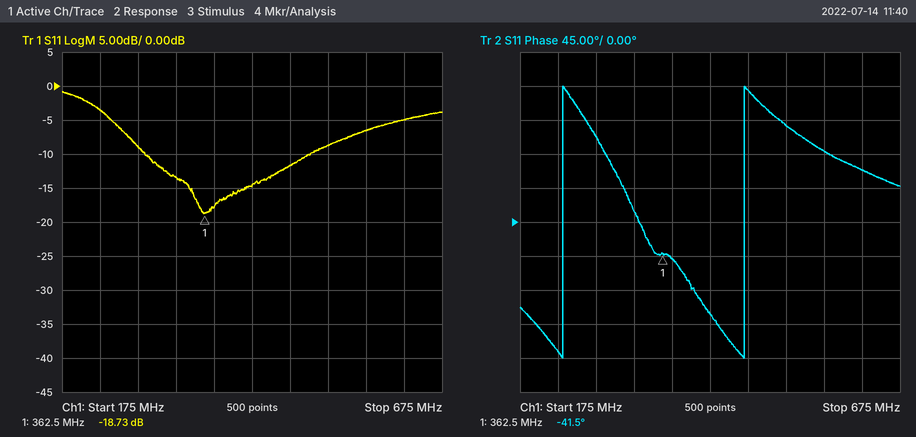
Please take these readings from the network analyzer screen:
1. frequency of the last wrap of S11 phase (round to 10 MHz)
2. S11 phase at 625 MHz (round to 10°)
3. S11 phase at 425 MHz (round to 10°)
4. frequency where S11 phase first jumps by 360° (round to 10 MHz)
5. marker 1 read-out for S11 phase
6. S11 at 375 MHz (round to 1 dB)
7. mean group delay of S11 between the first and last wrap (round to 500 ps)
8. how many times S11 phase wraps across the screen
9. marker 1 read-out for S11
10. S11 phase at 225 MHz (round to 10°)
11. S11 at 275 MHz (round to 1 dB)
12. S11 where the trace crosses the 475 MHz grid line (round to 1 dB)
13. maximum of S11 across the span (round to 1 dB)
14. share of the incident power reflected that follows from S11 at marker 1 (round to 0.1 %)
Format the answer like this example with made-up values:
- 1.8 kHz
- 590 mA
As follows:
- 470 MHz
- 70°
- -120°
- 230 MHz
- -41.5°
- -18 dB
- 4.0 ns
- 2
- -18.73 dB
- -170°
- -9 dB
- -12 dB
- -1 dB
- 1.3 %
